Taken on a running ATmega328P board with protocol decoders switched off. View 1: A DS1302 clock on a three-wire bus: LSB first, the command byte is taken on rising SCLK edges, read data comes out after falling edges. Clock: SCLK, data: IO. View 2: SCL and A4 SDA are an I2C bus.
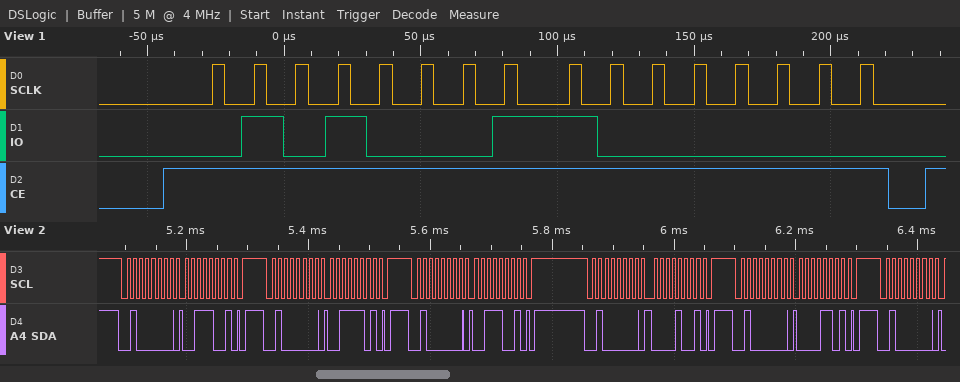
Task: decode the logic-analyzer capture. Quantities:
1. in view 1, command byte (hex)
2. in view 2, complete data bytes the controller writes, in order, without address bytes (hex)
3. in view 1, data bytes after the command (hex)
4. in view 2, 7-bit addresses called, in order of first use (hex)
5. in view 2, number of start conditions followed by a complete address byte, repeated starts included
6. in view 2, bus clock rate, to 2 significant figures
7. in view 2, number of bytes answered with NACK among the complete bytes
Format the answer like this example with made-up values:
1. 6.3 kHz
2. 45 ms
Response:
1. 0x8A
2. 39 3D 39 09 0D
3. 01
4. 0x20
5. 6
6. 100 kHz
7. 0
